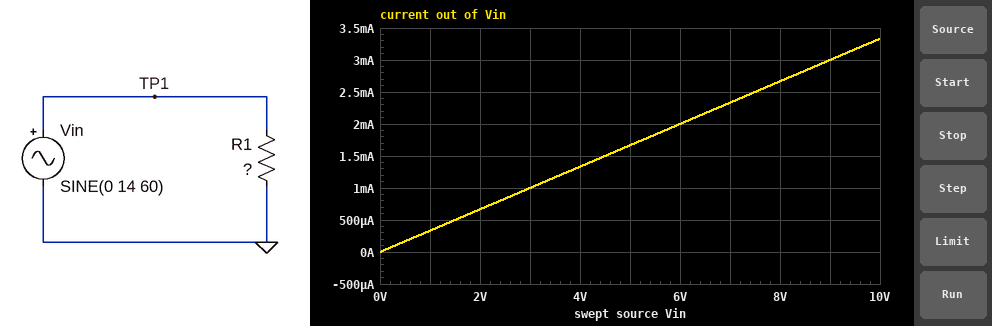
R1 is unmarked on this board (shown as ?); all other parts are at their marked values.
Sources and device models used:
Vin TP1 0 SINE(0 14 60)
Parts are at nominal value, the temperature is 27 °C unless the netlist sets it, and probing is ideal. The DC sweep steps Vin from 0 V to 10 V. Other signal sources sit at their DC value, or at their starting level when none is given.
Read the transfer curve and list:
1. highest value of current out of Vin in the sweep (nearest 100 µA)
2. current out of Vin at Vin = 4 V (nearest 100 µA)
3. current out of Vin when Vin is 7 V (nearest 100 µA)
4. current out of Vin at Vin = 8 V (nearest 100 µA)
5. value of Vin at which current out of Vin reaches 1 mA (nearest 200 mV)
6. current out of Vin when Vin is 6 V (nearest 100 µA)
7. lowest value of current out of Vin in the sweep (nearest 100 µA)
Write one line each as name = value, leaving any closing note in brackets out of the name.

highest value of current out of Vin in the sweep = 3.3 mA
current out of Vin at Vin = 4 V = 1.3 mA
current out of Vin when Vin is 7 V = 2.3 mA
current out of Vin at Vin = 8 V = 2.7 mA
value of Vin at which current out of Vin reaches 1 mA = 3.0 V
current out of Vin when Vin is 6 V = 2.0 mA
lowest value of current out of Vin in the sweep = 0 A
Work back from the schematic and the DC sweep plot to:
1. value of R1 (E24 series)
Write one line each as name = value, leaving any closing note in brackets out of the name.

value of R1 = 3 kΩ
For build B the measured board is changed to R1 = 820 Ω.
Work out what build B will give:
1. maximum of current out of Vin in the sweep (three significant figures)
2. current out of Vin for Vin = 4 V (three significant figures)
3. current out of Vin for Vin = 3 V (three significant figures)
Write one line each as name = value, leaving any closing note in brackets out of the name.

maximum of current out of Vin in the sweep = 12.2 mA
current out of Vin for Vin = 4 V = 4.88 mA
current out of Vin for Vin = 3 V = 3.66 mA
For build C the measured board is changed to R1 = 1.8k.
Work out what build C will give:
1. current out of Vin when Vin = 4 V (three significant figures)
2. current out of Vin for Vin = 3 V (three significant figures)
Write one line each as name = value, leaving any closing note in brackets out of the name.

current out of Vin when Vin = 4 V = 2.22 mA
current out of Vin for Vin = 3 V = 1.67 mA
